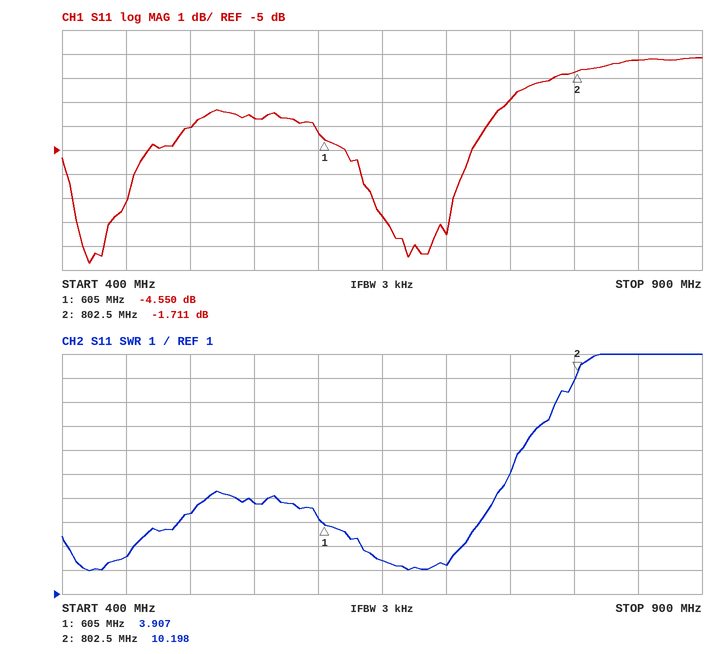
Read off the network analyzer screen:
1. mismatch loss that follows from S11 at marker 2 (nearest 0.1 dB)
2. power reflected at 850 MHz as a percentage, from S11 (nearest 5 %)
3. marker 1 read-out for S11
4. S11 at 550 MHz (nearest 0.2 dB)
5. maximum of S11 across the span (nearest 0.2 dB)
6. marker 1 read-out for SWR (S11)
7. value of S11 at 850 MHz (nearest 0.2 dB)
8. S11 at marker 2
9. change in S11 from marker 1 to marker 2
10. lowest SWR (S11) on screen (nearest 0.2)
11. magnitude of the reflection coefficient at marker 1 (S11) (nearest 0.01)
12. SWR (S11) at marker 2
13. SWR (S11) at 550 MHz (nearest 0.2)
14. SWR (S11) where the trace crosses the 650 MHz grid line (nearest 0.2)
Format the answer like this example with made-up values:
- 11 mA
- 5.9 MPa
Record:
- 4.9 dB
- 75 %
- -4.550 dB
- -3.6 dB
- -1.2 dB
- 3.907
- -1.2 dB
- -1.711 dB
- 2.839 dB
- 2.0
- 0.59
- 10.198
- 4.8
- 2.4
